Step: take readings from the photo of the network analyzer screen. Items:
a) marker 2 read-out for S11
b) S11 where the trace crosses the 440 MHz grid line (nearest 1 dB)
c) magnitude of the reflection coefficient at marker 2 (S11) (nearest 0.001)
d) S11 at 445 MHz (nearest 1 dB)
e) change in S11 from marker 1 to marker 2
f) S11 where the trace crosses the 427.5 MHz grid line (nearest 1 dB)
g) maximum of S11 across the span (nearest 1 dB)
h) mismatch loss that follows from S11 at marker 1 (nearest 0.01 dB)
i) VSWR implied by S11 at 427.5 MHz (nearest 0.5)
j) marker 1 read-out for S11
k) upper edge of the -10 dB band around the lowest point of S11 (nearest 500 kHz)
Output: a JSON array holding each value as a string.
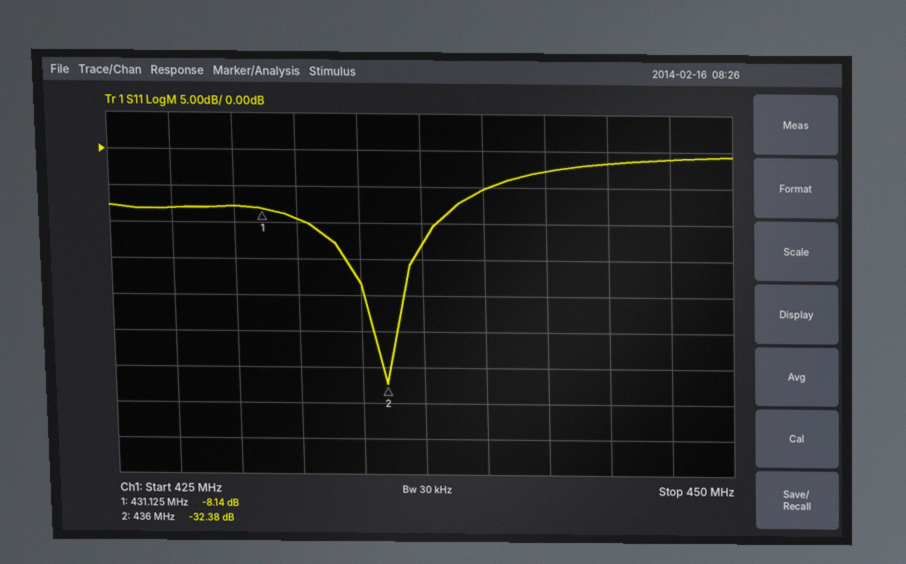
["-32.38 dB", "-5 dB", "0.024", "-2 dB", "-24.24 dB", "-8 dB", "-1 dB", "0.72 dB", "2.5", "-8.14 dB", "438.0 MHz"]
